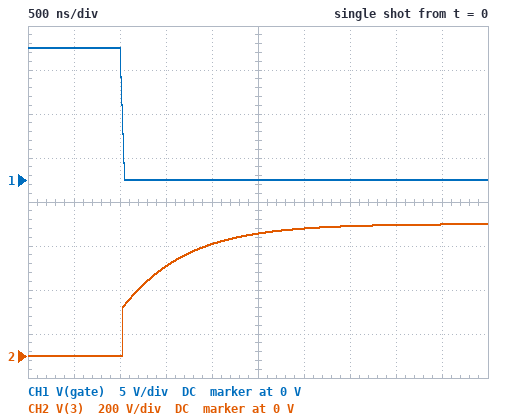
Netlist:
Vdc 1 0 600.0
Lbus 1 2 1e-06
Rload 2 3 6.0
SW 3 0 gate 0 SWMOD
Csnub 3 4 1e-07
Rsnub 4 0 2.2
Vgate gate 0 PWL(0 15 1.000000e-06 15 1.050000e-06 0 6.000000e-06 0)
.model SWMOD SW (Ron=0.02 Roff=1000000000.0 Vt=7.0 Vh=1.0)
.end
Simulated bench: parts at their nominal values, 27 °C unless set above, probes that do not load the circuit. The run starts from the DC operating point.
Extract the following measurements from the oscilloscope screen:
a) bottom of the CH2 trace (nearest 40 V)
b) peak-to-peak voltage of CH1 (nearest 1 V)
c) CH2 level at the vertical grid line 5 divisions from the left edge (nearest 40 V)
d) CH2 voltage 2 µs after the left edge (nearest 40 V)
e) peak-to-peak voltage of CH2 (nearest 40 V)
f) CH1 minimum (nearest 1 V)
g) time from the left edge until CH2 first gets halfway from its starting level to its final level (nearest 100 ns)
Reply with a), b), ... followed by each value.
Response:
a) 0 V
b) 15 V
c) 560 V
d) 520 V
e) 600 V
f) 0 V
g) 1.2 µs
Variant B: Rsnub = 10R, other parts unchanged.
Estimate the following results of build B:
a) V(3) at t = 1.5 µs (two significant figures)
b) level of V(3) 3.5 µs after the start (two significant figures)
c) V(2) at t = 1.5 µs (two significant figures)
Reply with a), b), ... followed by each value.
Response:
a) 460 V
b) 560 V
c) 620 V
